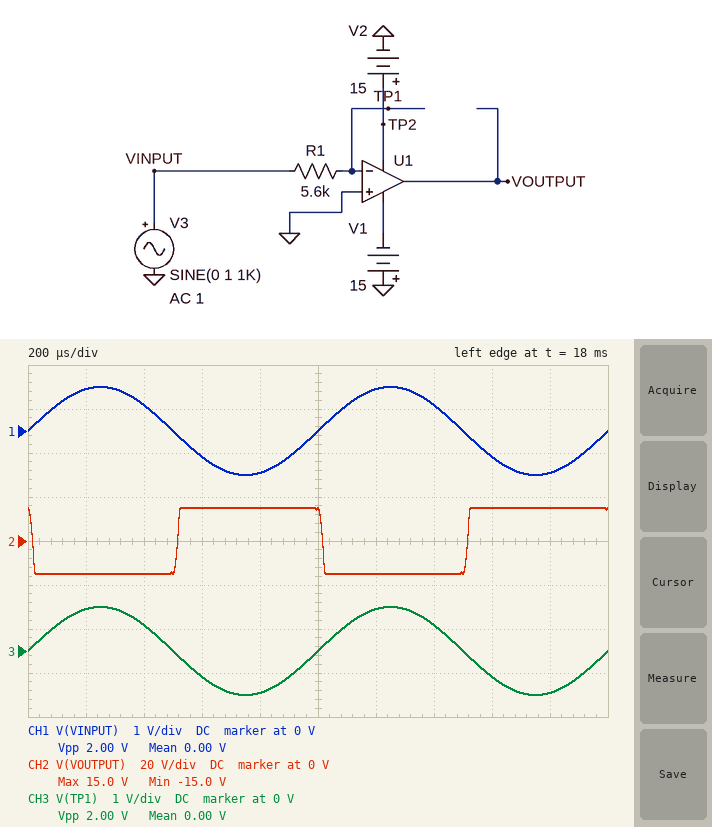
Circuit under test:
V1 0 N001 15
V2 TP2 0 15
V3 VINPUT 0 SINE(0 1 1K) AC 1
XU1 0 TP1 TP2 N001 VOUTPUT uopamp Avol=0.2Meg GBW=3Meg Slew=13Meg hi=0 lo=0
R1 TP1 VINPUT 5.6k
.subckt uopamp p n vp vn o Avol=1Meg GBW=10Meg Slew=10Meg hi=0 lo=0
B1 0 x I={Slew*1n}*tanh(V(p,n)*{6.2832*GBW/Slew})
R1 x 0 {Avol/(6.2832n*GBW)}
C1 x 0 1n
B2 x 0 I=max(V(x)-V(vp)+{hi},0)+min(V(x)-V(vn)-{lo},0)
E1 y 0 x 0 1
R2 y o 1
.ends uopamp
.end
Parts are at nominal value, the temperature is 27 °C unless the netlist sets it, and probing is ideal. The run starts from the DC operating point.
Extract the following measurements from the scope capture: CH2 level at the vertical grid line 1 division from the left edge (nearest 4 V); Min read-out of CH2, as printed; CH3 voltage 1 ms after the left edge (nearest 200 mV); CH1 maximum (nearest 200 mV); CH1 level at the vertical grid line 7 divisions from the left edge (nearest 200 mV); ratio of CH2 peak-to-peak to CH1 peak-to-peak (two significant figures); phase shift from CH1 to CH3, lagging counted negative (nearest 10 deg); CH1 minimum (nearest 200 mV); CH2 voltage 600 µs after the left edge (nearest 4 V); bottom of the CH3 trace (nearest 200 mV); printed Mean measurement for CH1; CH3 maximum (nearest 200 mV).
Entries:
-16 V
-15.0 V
0 V
1.0 V
600 mV
15
0 deg
-1.0 V
16 V
-1.0 V
0.00 V
1.0 V
